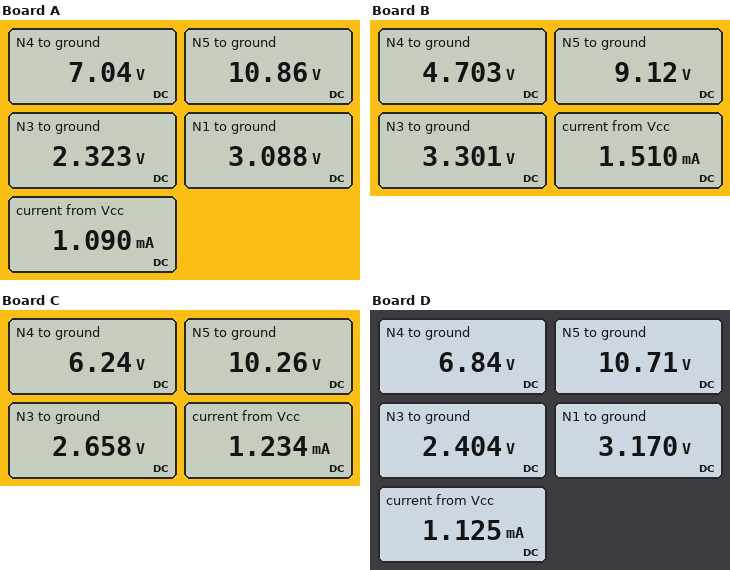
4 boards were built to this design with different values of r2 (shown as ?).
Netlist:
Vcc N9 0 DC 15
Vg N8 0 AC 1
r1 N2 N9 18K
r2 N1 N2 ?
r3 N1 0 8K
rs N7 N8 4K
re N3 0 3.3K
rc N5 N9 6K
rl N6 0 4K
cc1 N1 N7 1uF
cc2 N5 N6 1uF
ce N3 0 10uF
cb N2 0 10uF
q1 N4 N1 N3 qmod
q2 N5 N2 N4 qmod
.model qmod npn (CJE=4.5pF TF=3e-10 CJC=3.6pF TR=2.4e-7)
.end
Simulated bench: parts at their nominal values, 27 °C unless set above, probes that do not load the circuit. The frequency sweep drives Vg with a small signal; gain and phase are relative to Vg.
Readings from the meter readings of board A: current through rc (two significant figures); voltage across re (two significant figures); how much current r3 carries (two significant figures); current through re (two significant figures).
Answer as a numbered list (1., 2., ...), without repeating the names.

1. 690 µA
2. 2.3 V
3. 390 µA
4. 700 µA
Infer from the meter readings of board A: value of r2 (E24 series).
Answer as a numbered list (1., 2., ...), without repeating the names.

1. 12 kΩ
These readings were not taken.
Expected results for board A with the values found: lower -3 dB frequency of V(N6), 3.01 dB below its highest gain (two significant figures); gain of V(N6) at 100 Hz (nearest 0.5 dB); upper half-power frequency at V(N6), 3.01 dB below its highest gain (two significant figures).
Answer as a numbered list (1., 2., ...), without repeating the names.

1. 290 Hz
2. 17.0 dB
3. 5.7 MHz
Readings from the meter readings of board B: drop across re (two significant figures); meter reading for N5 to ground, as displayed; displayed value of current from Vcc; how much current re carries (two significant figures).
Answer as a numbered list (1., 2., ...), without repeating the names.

1. 3.3 V
2. 9.12 V
3. 1.510 mA
4. 1.0 mA
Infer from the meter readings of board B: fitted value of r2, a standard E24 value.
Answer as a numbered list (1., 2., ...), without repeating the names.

1. 2.7 kΩ
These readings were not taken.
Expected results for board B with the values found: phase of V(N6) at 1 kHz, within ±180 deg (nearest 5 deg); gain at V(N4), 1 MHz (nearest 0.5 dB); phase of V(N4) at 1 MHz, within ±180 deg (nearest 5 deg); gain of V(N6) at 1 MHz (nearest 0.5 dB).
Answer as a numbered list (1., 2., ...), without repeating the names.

1. -155 deg
2. -13.0 dB
3. 170 deg
4. 26.0 dB
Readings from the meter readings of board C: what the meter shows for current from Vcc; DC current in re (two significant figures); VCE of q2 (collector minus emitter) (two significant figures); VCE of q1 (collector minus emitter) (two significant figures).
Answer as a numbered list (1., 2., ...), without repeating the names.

1. 1.234 mA
2. 810 µA
3. 4.0 V
4. 3.6 V
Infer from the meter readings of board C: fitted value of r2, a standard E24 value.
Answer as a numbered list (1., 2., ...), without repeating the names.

1. 8.2 kΩ
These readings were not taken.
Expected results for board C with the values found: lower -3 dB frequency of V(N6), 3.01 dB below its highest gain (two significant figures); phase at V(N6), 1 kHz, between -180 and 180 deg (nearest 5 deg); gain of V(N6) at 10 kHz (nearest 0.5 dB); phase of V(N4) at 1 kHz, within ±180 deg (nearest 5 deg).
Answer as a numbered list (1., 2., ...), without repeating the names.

1. 320 Hz
2. -160 deg
3. 27.0 dB
4. -160 deg
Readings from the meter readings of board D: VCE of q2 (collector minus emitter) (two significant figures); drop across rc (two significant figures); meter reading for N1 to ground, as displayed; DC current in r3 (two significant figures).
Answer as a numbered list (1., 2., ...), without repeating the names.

1. 3.9 V
2. 4.3 V
3. 3.170 V
4. 400 µA
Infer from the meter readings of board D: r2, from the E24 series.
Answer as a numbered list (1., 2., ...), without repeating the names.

1. 11 kΩ
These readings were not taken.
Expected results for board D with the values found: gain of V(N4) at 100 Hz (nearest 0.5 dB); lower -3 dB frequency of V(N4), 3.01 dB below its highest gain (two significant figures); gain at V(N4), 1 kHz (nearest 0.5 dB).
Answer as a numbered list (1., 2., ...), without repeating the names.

1. -19.0 dB
2. 290 Hz
3. -10.0 dB
